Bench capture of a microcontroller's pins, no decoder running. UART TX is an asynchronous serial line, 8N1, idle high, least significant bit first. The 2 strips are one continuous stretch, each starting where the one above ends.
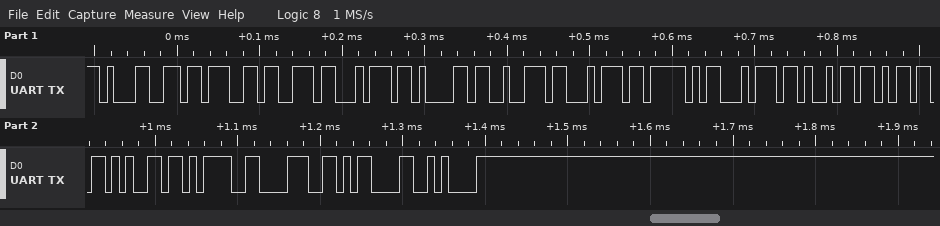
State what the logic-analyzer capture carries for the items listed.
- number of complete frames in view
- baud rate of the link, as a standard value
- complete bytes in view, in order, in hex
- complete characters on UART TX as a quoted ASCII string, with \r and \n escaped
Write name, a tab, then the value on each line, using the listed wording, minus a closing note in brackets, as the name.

number of complete frames in view	16
baud rate of the link, as a standard value	115200 baud
complete bytes in view, in order, in hex	31 3B 73 74 61 72 74 5F 74 69 6D 65 3D 38 0D 0A
complete characters on UART TX as a quoted ASCII string, with \r and \n escaped	"1;start_time=8\r\n"
